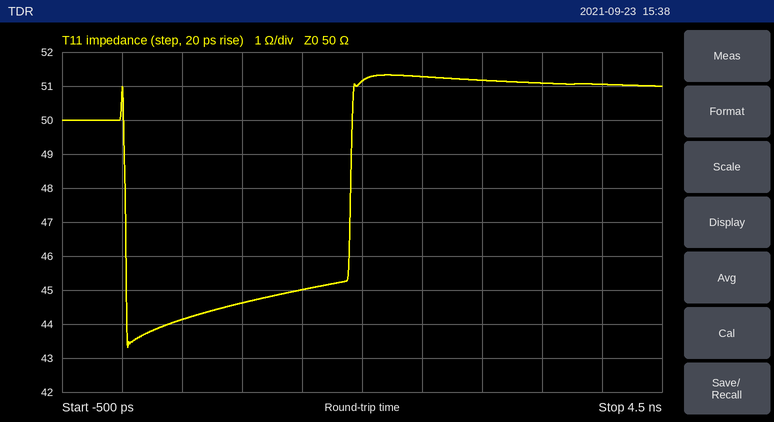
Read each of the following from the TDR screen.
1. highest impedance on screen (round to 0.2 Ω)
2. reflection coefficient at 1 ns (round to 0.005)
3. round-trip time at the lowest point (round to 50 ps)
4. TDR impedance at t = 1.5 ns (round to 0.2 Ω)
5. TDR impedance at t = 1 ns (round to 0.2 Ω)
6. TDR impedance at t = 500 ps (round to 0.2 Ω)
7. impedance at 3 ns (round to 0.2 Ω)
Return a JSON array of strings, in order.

["51.4 Ω", "-0.055", "50 ps", "45.0 Ω", "44.6 Ω", "44.2 Ω", "51.2 Ω"]
